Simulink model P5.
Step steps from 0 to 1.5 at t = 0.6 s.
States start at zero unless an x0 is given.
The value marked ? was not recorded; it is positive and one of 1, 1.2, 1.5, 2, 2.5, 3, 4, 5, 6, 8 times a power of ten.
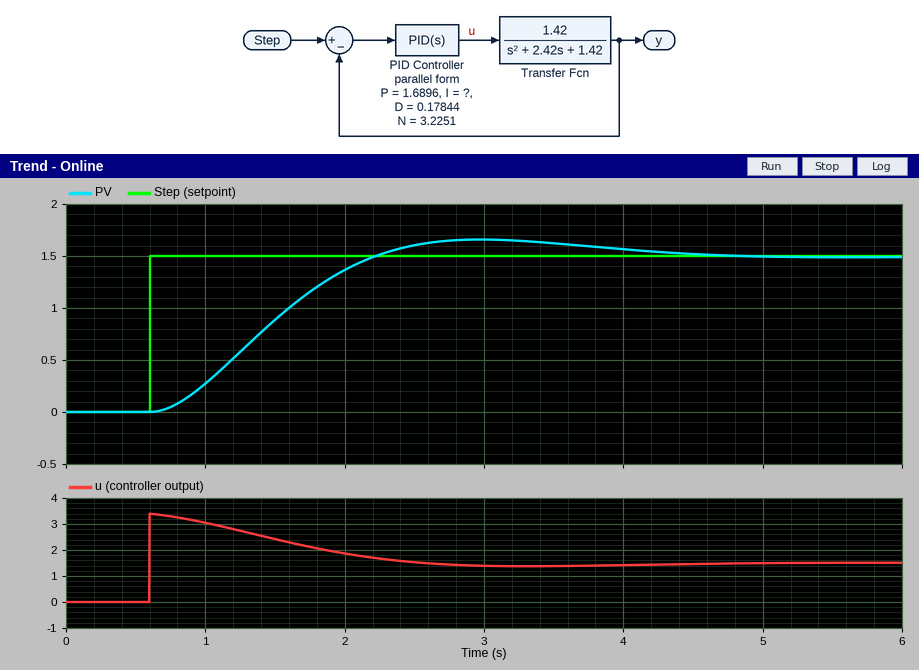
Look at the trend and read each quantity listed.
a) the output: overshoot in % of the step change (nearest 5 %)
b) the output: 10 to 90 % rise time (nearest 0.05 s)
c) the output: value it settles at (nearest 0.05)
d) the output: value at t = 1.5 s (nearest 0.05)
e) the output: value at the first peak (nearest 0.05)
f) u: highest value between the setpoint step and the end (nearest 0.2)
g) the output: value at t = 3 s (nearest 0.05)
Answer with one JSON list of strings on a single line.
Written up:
["10 %", "1.10 s", "1.50", "0.90", "1.65", "3.4", "1.65"]
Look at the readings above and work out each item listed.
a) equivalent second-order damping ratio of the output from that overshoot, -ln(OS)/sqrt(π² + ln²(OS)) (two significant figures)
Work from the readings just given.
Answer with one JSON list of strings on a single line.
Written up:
["0.59"]
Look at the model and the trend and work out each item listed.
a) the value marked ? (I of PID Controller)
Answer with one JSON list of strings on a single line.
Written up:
["1.5"]
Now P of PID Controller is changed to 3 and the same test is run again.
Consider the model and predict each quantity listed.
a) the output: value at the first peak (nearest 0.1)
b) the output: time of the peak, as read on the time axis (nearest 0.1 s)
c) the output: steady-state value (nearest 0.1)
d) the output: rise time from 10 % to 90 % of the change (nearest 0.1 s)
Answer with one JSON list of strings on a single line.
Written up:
["1.6", "2.2 s", "1.5", "0.8 s"]
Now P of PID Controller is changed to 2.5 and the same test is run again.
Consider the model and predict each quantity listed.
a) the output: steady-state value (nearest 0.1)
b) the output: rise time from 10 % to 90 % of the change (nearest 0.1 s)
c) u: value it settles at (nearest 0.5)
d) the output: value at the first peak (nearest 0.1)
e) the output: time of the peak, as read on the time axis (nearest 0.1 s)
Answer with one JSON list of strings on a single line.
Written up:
["1.5", "0.9 s", "1.5", "1.6", "2.4 s"]
